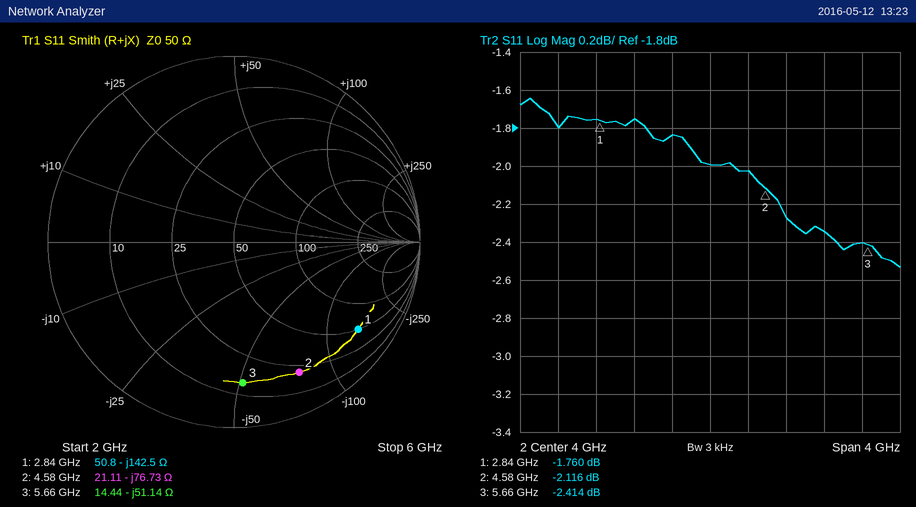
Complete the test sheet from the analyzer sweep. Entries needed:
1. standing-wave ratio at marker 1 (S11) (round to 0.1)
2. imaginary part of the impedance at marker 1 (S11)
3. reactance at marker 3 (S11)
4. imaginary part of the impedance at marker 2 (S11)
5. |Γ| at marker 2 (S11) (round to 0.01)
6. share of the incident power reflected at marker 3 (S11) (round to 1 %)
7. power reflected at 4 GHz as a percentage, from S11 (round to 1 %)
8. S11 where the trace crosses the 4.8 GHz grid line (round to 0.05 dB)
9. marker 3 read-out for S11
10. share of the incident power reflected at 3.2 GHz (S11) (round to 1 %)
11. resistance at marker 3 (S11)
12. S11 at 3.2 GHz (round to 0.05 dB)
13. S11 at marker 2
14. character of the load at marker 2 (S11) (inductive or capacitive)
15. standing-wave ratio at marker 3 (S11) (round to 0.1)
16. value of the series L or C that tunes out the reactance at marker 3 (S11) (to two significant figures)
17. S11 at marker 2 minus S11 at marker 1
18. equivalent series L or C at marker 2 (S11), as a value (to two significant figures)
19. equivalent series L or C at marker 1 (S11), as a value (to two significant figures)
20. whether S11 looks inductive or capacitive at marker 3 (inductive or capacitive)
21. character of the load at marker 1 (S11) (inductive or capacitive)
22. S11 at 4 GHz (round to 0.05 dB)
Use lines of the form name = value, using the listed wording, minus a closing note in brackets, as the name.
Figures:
standing-wave ratio at marker 1 (S11) = 9.9
imaginary part of the impedance at marker 1 = -142.5 Ω
reactance at marker 3 = -51.14 Ω
imaginary part of the impedance at marker 2 = -76.73 Ω
|Γ| at marker 2 (S11) = 0.78
share of the incident power reflected at marker 3 (S11) = 57 %
power reflected at 4 GHz as a percentage, from S11 = 63 %
S11 where the trace crosses the 4.8 GHz grid line = -2.25 dB
marker 3 read-out for S11 = -2.414 dB
share of the incident power reflected at 3.2 GHz (S11) = 67 %
resistance at marker 3 = 14.44 Ω
S11 at 3.2 GHz = -1.75 dB
S11 at marker 2 = -2.116 dB
character of the load at marker 2 (S11) = capacitive
standing-wave ratio at marker 3 (S11) = 7.2
value of the series L or C that tunes out the reactance at marker 3 (S11) = 1.4 nH
S11 at marker 2 minus S11 at marker 1 = -0.356 dB
equivalent series L or C at marker 2 (S11), as a value = 450 fF
equivalent series L or C at marker 1 (S11), as a value = 390 fF
whether S11 looks inductive or capacitive at marker 3 = capacitive
character of the load at marker 1 (S11) = capacitive
S11 at 4 GHz = -2.00 dB
